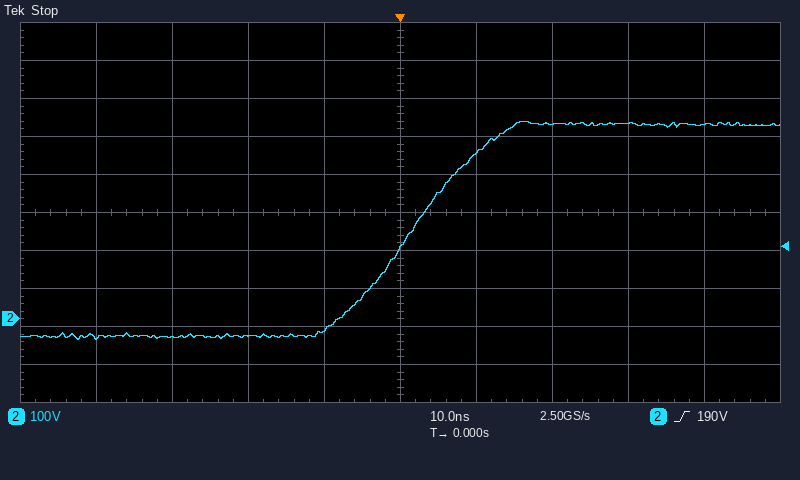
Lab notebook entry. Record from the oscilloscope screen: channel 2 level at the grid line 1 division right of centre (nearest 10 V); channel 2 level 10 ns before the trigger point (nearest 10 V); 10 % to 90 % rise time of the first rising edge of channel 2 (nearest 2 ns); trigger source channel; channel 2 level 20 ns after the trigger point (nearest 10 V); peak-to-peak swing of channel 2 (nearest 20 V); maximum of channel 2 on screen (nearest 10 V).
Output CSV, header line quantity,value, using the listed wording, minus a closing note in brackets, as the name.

quantity,value
channel 2 level at the grid line 1 division right of centre,440 V
channel 2 level 10 ns before the trigger point,-30 V
10 % to 90 % rise time of the first rising edge of channel 2,18 ns
trigger source channel,channel 2
channel 2 level 20 ns after the trigger point,510 V
peak-to-peak swing of channel 2,580 V
maximum of channel 2 on screen,520 V
